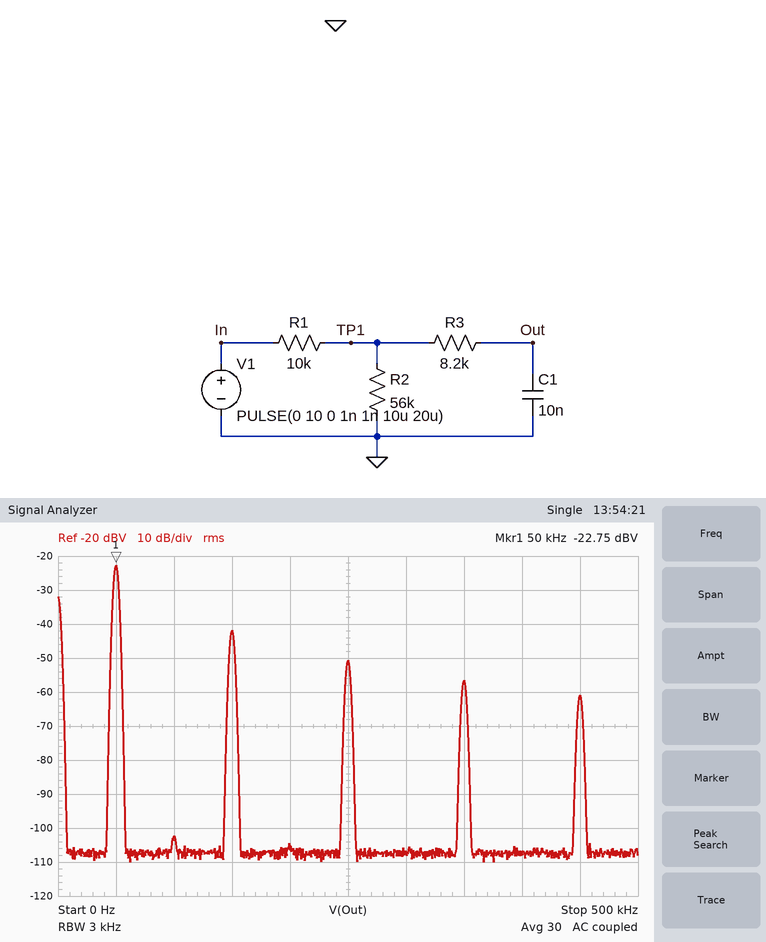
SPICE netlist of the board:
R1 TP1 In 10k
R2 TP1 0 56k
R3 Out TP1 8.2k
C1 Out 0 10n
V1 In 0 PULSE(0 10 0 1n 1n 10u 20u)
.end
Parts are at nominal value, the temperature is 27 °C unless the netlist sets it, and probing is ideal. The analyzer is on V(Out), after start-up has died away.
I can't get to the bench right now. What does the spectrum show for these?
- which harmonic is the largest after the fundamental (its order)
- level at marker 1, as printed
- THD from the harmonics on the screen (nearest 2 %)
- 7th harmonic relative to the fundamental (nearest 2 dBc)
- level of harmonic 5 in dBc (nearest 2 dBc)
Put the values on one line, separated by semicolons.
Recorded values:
3; -22.75 dBV; 12 %; -34 dBc; -28 dBc
